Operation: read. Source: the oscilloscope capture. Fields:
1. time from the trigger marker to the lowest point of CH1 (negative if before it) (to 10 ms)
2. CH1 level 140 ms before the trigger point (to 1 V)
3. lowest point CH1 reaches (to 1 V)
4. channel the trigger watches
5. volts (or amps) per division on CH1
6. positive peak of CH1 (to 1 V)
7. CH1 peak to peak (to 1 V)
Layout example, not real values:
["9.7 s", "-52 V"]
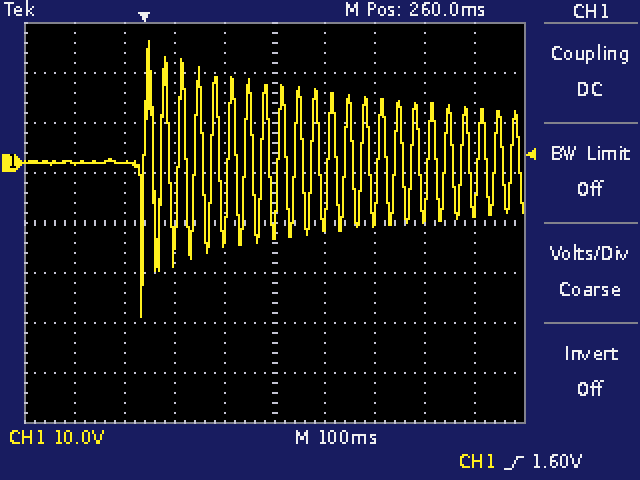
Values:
["-10 ms", "0 V", "-31 V", "CH1", "10 V", "24 V", "55 V"]
